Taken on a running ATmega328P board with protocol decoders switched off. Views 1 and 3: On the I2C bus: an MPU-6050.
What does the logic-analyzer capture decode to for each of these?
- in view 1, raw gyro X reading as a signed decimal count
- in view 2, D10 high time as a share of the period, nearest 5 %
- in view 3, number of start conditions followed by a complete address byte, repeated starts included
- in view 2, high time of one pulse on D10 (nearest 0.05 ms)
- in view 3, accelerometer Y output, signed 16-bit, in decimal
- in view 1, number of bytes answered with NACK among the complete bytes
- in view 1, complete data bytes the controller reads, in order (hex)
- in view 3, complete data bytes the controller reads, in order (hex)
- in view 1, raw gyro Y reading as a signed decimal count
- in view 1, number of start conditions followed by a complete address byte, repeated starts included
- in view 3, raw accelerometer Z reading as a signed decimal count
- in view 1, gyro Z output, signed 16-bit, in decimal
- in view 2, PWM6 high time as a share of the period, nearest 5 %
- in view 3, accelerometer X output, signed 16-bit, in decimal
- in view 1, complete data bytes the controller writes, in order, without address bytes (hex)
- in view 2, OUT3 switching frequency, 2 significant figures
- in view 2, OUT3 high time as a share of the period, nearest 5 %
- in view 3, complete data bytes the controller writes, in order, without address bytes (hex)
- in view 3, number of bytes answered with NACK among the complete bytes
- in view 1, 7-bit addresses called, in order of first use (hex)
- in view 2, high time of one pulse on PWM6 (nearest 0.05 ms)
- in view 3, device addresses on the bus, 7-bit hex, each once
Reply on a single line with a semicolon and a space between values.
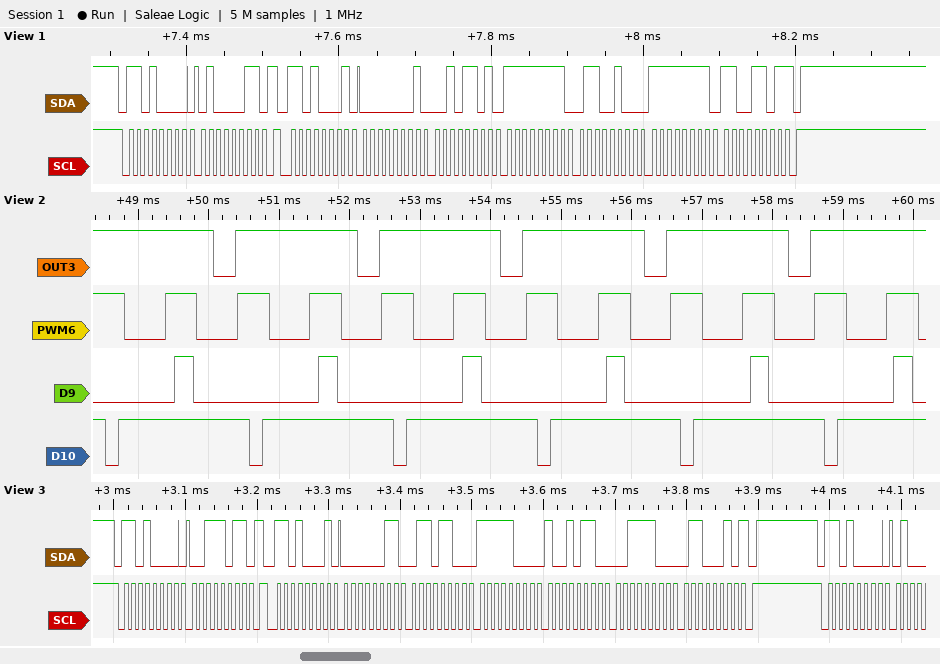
301; 90 %; 3; 1.85 ms; -1898; 1; 01 2D FF 64 FF CD; 03 6C F8 96 3C 62; -156; 2; 15458; -51; 45 %; 876; 43; 490 Hz; 85 %; 3B; 1; 0x68; 0.45 ms; 0x68
